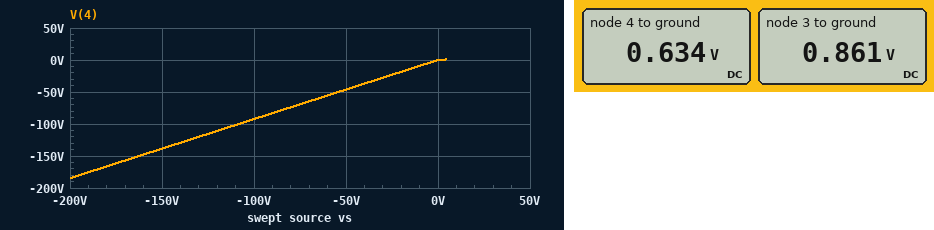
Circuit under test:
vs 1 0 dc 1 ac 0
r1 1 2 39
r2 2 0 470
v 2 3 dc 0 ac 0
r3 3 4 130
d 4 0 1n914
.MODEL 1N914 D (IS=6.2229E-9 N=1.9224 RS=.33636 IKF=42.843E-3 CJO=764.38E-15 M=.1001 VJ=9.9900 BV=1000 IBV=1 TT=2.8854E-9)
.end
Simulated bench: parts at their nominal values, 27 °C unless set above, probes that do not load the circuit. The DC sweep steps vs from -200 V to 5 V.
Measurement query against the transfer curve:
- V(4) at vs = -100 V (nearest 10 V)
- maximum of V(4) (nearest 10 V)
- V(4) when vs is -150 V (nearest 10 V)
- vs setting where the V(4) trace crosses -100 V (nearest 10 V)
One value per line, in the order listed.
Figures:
-90 V
0 V
-140 V
-110 V
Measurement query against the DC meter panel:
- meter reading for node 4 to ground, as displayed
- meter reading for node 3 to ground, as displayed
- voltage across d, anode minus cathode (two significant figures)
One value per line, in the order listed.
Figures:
0.634 V
0.861 V
630 mV
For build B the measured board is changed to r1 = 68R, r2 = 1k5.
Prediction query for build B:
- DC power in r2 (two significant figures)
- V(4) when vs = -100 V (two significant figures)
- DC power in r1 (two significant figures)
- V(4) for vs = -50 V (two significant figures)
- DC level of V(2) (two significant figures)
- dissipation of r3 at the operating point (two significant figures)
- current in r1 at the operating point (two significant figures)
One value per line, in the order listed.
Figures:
480 µW
-96 V
340 µW
-48 V
850 mV
360 µW
2.2 mA
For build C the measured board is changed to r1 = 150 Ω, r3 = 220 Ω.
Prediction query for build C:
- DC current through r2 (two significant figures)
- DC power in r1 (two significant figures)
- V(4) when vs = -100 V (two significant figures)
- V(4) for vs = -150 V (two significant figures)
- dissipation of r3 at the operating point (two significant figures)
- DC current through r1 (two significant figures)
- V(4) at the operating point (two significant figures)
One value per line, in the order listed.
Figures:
1.5 mA
620 µW
-76 V
-110 V
68 µW
2.0 mA
570 mV
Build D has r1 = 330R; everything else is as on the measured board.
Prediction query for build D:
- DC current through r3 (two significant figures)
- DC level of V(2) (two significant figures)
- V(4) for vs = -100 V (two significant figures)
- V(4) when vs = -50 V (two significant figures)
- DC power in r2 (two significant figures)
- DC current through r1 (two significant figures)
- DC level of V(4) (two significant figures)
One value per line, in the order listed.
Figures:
210 µA
550 mV
-59 V
-29 V
640 µW
1.4 mA
520 mV
